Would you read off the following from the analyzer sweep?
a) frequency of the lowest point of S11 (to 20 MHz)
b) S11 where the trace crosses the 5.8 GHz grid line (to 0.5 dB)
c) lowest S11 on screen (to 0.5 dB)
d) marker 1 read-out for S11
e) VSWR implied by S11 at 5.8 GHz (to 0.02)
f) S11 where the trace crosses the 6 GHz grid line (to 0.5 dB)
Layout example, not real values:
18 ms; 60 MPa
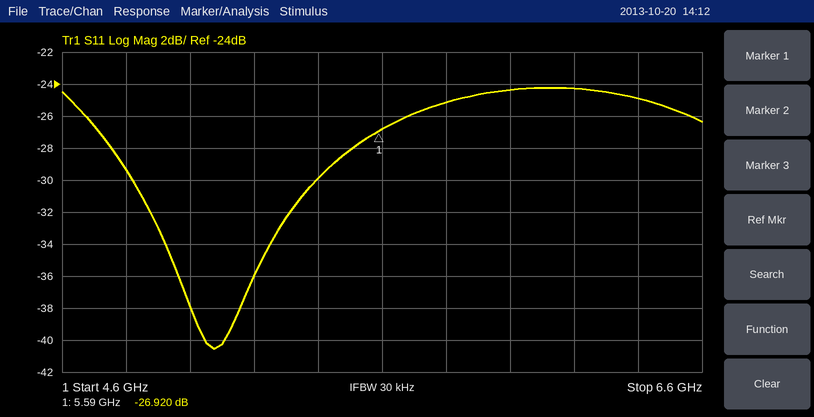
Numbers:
5.08 GHz; -25.0 dB; -40.5 dB; -26.920 dB; 1.12; -24.5 dB
